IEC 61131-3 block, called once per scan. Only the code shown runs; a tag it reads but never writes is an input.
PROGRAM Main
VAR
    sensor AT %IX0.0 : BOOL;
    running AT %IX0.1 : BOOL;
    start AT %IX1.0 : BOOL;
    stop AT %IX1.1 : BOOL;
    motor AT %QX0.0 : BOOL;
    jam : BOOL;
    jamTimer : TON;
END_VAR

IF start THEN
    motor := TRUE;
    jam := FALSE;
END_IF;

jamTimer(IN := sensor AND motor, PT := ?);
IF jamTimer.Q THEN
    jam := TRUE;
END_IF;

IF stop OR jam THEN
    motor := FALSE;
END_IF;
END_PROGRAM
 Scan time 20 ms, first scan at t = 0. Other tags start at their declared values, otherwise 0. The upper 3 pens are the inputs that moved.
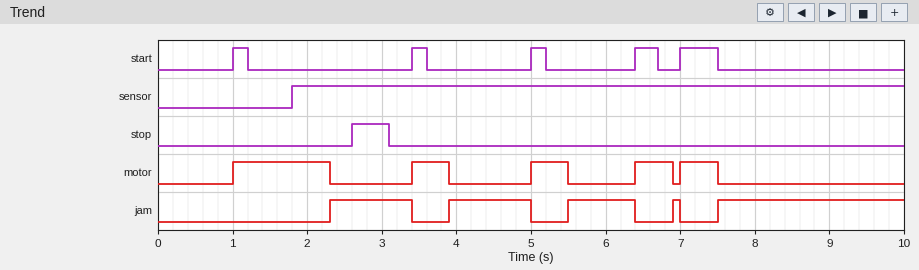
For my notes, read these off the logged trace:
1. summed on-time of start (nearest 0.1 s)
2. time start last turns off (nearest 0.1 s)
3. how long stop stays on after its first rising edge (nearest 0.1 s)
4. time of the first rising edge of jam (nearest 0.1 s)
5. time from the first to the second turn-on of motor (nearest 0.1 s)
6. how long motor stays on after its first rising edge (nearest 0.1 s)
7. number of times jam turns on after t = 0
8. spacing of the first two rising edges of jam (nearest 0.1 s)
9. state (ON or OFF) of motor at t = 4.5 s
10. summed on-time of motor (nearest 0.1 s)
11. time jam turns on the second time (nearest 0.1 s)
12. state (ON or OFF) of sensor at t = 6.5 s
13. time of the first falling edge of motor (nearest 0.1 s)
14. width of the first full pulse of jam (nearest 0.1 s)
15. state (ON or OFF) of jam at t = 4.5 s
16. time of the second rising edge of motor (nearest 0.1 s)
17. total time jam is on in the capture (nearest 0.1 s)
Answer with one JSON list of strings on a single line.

["1.4 s", "7.5 s", "0.5 s", "2.3 s", "2.4 s", "1.3 s", "5", "1.6 s", "OFF", "3.3 s", "3.9 s", "ON", "2.3 s", "1.1 s", "ON", "3.4 s", "5.7 s"]
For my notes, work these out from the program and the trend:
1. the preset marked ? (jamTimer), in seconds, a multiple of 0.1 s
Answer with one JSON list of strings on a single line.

["0.5 s"]
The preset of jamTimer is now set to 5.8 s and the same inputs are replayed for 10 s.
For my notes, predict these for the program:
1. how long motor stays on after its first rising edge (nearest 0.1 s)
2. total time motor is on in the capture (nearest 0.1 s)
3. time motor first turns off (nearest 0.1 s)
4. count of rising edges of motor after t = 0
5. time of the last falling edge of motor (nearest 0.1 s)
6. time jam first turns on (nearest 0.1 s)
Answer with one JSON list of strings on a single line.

["1.6 s", "7.4 s", "2.6 s", "2", "9.2 s", "9.2 s"]
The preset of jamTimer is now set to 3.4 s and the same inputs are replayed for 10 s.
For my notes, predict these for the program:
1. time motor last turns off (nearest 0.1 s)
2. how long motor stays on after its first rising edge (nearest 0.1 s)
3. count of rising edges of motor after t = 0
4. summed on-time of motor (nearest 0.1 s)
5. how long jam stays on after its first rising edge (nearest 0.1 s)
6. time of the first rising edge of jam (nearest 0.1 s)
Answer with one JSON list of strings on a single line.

["6.8 s", "1.6 s", "3", "8.0 s", "0.2 s", "6.8 s"]
